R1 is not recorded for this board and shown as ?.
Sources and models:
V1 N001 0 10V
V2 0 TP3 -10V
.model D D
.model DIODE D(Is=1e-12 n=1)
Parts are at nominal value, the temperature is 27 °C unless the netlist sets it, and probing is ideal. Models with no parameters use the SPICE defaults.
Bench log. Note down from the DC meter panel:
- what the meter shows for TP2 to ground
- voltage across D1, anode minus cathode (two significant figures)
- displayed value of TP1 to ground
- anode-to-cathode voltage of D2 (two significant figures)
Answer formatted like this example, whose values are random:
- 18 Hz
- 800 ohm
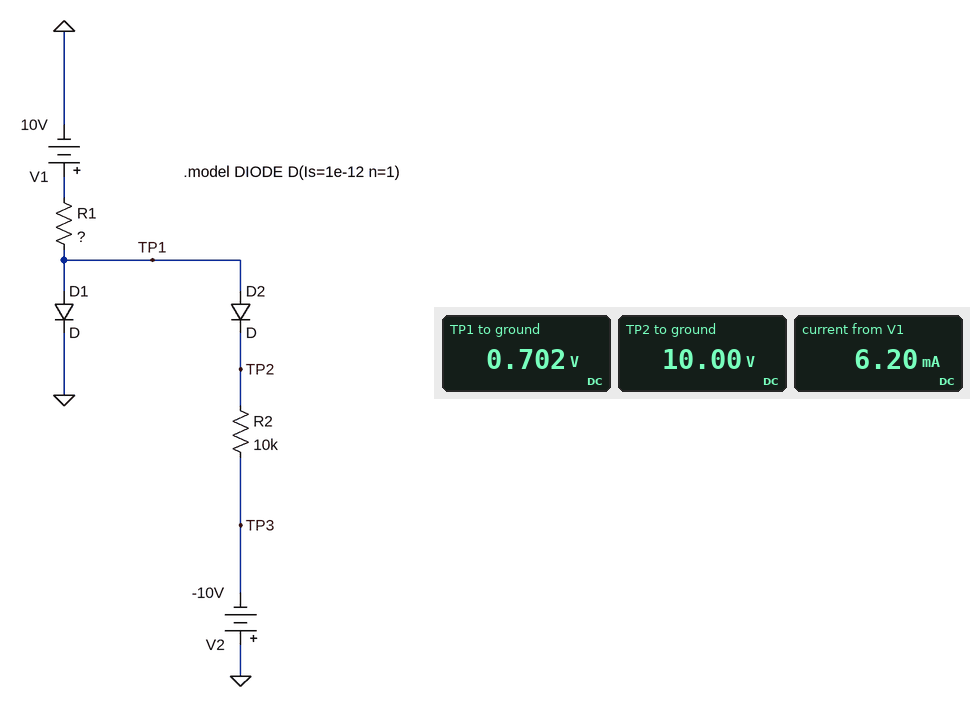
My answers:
- 10.00 V
- 700 mV
- 0.702 V
- -9.3 V
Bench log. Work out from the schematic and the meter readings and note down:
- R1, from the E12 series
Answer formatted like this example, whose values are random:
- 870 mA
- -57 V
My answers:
- 1.5 kΩ
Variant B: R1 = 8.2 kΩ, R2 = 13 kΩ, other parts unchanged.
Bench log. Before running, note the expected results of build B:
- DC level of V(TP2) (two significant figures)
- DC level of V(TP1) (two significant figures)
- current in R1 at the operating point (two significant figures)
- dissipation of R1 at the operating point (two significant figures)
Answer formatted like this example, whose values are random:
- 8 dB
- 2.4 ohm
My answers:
- 10 V
- 660 mV
- 1.1 mA
- 11 mW
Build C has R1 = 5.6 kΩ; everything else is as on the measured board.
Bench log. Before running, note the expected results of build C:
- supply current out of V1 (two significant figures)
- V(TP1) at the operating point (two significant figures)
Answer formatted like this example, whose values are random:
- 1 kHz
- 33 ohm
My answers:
- 1.7 mA
- 670 mV
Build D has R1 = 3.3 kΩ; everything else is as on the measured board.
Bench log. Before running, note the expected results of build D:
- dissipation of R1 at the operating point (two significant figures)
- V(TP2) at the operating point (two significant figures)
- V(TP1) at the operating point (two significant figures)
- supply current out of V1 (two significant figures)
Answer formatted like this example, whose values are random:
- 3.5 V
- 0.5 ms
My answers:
- 26 mW
- 10 V
- 680 mV
- 2.8 mA
